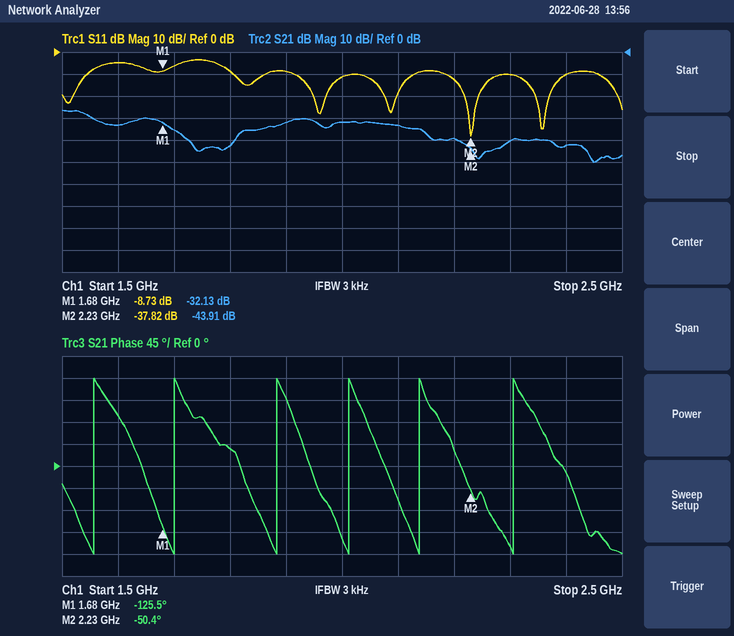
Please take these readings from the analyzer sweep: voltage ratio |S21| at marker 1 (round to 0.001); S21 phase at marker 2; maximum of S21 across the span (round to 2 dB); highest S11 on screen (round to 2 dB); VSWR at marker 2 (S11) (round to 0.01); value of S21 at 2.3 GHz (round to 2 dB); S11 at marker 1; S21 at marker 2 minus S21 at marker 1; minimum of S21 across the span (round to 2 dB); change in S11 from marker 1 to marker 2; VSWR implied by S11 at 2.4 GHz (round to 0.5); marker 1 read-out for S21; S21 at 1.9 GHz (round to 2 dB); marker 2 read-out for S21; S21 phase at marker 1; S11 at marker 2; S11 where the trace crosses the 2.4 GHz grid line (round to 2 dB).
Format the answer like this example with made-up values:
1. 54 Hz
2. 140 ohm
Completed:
1. 0.025
2. -50.4°
3. -26 dB
4. -4 dB
5. 1.03
6. -40 dB
7. -8.73 dB
8. -11.78 dB
9. -50 dB
10. -29.09 dB
11. 2.0
12. -32.13 dB
13. -32 dB
14. -43.91 dB
15. -125.5°
16. -37.82 dB
17. -10 dB
